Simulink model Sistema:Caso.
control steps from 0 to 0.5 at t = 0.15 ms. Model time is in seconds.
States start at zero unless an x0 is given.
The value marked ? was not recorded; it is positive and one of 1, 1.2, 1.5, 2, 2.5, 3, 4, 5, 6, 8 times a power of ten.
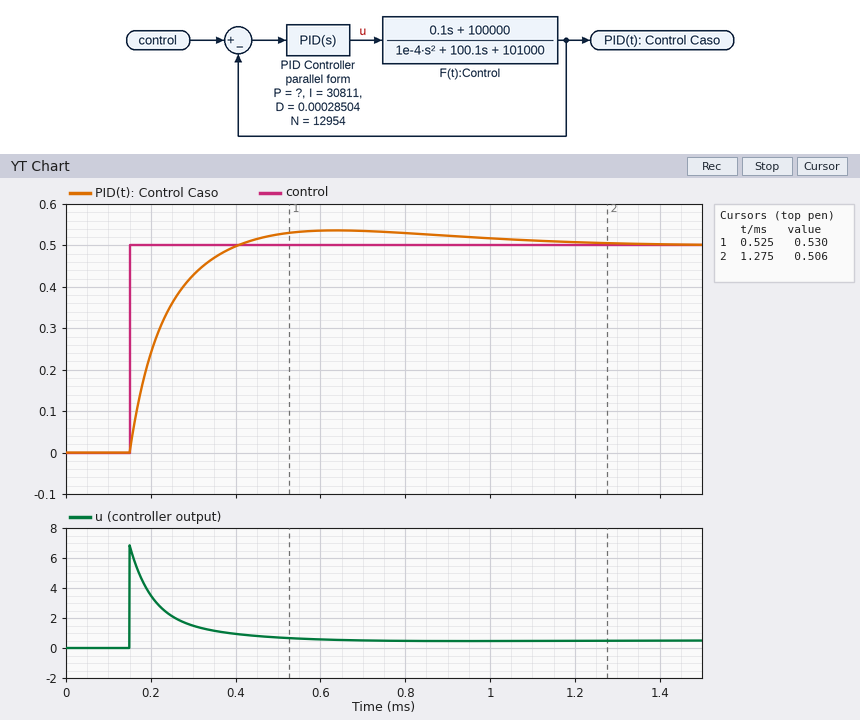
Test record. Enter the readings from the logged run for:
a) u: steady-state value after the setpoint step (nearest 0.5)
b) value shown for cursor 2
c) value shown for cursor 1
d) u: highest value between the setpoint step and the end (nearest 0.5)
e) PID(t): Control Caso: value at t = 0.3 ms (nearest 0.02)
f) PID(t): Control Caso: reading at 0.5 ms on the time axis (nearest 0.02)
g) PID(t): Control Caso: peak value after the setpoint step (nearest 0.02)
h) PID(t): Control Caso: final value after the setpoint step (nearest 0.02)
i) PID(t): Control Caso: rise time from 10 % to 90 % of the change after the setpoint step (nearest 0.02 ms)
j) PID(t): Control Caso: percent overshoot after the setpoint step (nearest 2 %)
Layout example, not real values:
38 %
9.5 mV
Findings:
0.5
0.506
0.530
7.0
0.42
0.52
0.54
0.50
0.16 ms
8 %
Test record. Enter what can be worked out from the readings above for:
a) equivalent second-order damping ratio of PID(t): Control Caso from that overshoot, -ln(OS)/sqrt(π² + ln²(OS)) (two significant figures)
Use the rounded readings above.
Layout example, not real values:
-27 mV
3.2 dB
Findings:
0.63
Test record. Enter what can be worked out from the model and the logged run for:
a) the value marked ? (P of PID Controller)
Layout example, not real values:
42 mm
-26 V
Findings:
10
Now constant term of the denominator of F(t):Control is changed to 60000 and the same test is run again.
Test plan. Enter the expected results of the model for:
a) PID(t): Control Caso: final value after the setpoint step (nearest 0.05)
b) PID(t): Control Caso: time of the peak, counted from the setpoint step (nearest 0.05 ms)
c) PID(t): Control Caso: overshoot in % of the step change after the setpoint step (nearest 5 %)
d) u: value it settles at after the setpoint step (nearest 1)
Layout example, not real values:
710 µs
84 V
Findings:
0.50
0.45 ms
10 %
0
